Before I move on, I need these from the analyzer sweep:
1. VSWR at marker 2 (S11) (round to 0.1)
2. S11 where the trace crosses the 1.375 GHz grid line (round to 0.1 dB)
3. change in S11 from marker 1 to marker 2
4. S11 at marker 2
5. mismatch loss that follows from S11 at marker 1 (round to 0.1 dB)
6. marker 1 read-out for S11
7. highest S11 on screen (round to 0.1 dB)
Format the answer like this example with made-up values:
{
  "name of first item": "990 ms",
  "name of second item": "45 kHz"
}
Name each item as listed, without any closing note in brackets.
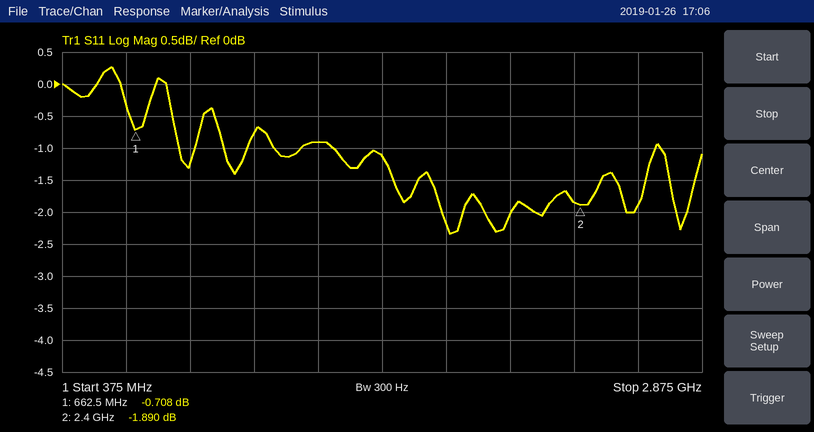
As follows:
{
  "VSWR at marker 2 (S11)": "9.2",
  "S11 where the trace crosses the 1.375 GHz grid line": "-0.9 dB",
  "change in S11 from marker 1 to marker 2": "-1.182 dB",
  "S11 at marker 2": "-1.890 dB",
  "mismatch loss that follows from S11 at marker 1": "8.2 dB",
  "marker 1 read-out for S11": "-0.708 dB",
  "highest S11 on screen": "0.3 dB"
}
